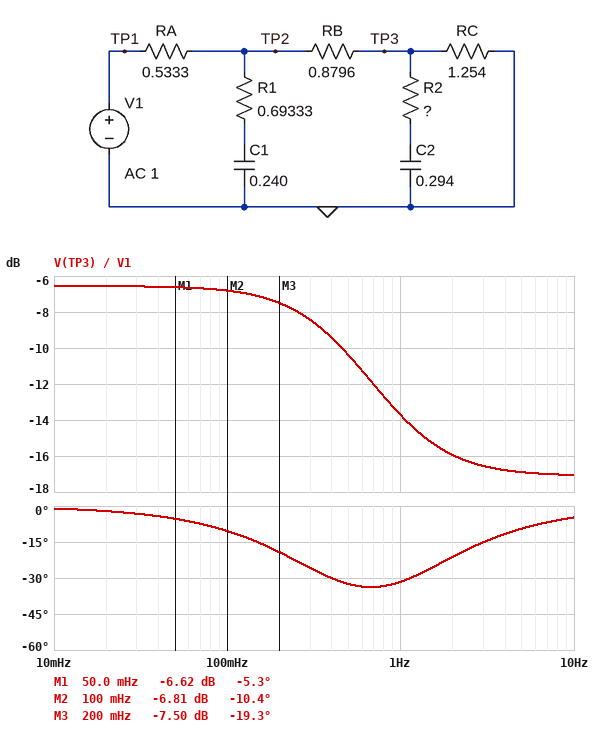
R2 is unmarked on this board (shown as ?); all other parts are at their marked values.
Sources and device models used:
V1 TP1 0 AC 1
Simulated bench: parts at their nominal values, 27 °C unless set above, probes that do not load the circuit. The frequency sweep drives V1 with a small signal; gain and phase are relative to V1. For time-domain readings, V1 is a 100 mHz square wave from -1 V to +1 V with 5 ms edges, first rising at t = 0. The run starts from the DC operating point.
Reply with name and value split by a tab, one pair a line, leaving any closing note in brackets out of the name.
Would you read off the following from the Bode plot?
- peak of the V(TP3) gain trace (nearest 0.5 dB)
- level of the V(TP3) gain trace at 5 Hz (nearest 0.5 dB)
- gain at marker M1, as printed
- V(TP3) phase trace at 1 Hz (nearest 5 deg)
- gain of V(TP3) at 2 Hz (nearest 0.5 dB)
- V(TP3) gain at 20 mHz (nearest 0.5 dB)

peak of the V(TP3) gain trace	-6.5 dB
level of the V(TP3) gain trace at 5 Hz	-17.0 dB
gain at marker M1, as printed	-6.62 dB
V(TP3) phase trace at 1 Hz	-30 deg
gain of V(TP3) at 2 Hz	-16.0 dB
V(TP3) gain at 20 mHz	-6.5 dB
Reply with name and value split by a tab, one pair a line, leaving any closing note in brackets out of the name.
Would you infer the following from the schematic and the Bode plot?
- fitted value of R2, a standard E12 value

fitted value of R2, a standard E12 value	0.56 Ω
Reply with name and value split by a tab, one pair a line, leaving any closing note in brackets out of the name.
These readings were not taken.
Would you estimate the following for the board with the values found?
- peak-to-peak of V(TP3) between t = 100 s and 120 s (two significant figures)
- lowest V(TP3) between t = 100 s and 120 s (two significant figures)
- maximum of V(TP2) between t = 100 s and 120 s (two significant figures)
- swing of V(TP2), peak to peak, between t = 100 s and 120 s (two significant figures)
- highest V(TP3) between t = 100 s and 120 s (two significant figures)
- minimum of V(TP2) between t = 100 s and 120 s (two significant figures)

peak-to-peak of V(TP3) between t = 100 s and 120 s	940 mV
lowest V(TP3) between t = 100 s and 120 s	-470 mV
maximum of V(TP2) between t = 100 s and 120 s	800 mV
swing of V(TP2), peak to peak, between t = 100 s and 120 s	1.6 V
highest V(TP3) between t = 100 s and 120 s	470 mV
minimum of V(TP2) between t = 100 s and 120 s	-800 mV
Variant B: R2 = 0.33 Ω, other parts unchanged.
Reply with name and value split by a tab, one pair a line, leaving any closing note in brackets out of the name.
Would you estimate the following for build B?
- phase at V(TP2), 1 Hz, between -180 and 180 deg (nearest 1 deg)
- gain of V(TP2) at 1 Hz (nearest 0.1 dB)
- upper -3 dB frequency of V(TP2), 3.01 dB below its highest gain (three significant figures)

phase at V(TP2), 1 Hz, between -180 and 180 deg	-15 deg
gain of V(TP2) at 1 Hz	-5.4 dB
upper -3 dB frequency of V(TP2), 3.01 dB below its highest gain	801 mHz
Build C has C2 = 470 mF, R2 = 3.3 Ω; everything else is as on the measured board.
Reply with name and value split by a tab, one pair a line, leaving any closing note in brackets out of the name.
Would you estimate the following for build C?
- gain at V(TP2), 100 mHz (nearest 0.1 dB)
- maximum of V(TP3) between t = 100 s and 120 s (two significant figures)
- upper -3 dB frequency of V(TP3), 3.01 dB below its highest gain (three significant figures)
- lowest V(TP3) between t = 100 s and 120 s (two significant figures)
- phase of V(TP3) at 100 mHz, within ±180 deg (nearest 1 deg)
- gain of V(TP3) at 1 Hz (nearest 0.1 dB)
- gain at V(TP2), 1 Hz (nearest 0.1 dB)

gain at V(TP2), 100 mHz	-2.2 dB
maximum of V(TP3) between t = 100 s and 120 s	460 mV
upper -3 dB frequency of V(TP3), 3.01 dB below its highest gain	564 mHz
lowest V(TP3) between t = 100 s and 120 s	-460 mV
phase of V(TP3) at 100 mHz, within ±180 deg	-9 deg
gain of V(TP3) at 1 Hz	-10.7 dB
gain at V(TP2), 1 Hz	-4.8 dB
